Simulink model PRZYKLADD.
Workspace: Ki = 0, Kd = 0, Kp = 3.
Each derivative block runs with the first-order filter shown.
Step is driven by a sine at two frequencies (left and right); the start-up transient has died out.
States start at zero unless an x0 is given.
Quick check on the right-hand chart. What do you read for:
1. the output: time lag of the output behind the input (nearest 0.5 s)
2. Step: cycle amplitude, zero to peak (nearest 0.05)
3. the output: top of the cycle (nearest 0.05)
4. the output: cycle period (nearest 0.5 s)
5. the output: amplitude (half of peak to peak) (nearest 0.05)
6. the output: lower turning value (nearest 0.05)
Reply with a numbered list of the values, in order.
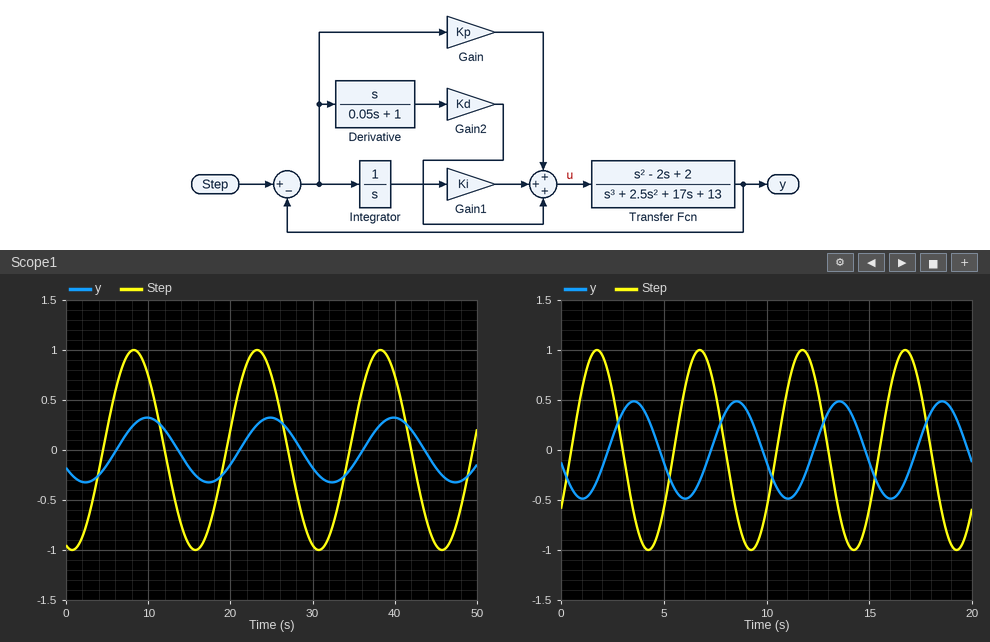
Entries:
1. 2.0 s
2. 1.00
3. 0.50
4. 5.0 s
5. 0.50
6. -0.50
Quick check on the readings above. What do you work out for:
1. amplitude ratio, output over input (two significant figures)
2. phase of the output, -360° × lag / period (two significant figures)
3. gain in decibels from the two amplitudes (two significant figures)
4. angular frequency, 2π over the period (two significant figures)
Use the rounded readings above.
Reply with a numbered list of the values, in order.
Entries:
1. 0.50
2. -140°
3. -6.0 dB
4. 1.3 rad/s
